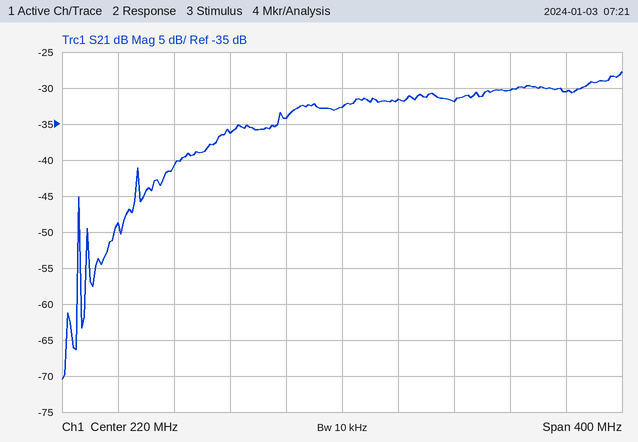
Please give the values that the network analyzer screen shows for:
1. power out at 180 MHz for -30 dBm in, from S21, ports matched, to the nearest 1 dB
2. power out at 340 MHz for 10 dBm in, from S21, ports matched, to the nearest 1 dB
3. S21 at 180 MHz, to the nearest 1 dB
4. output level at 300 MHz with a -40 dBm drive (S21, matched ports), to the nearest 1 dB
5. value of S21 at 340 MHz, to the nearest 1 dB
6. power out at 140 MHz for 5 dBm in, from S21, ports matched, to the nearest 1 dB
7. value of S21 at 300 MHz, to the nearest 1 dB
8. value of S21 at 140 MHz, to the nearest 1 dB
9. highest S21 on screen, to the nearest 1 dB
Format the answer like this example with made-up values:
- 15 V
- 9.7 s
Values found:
- -64 dBm
- -20 dBm
- -34 dB
- -72 dBm
- -30 dB
- -31 dBm
- -32 dB
- -36 dB
- -28 dB
